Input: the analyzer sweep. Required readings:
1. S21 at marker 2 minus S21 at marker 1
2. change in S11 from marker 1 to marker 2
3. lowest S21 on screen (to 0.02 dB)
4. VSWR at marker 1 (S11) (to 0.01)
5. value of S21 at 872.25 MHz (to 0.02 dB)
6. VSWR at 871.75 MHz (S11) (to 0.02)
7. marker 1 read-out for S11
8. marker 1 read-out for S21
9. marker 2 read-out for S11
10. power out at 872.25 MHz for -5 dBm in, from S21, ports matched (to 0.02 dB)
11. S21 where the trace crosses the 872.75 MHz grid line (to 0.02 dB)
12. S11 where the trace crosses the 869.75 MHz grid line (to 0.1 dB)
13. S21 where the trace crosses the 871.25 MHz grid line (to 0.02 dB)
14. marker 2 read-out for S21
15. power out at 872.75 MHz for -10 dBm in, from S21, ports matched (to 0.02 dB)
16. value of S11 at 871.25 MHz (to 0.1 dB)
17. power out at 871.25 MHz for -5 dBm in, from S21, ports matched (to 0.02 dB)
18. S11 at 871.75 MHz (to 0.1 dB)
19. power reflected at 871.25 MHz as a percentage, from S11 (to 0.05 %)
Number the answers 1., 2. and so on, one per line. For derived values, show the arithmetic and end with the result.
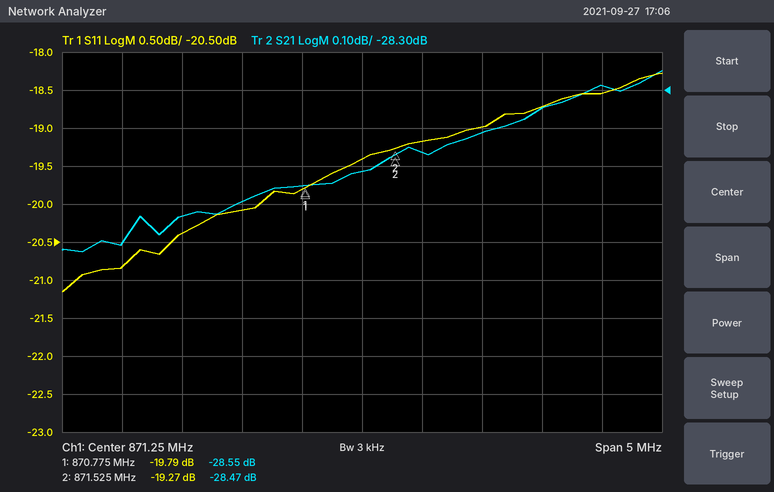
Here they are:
1. -28.47 − (-28.55) = 0.08 dB
2. -19.27 − (-19.79) = 0.52 dB
3. -28.72 dB
4. (1 + 0.1024)/(1 − 0.1024) ≈ 1.23
5. -28.42 dB
6. |Γ| = 10^(-19.2/20) = 0.1096; VSWR = (1 + 0.1096)/(1 − 0.1096) ≈ 1.25, so 1.24 to the nearest 0.02
7. -19.79 dB
8. -28.55 dB
9. -19.27 dB
10. -5 dBm + (-28.42 dB) = -33.42 dBm
11. -28.34 dB
12. -20.4 dB
13. -28.52 dB
14. -28.47 dB
15. -10 dBm + (-28.34 dB) = -38.34 dBm
16. -19.4 dB
17. -5 dBm + (-28.52 dB) = -33.52 dBm
18. -19.2 dB
19. 10^(-19.4/10) ≈ 1.15 %
